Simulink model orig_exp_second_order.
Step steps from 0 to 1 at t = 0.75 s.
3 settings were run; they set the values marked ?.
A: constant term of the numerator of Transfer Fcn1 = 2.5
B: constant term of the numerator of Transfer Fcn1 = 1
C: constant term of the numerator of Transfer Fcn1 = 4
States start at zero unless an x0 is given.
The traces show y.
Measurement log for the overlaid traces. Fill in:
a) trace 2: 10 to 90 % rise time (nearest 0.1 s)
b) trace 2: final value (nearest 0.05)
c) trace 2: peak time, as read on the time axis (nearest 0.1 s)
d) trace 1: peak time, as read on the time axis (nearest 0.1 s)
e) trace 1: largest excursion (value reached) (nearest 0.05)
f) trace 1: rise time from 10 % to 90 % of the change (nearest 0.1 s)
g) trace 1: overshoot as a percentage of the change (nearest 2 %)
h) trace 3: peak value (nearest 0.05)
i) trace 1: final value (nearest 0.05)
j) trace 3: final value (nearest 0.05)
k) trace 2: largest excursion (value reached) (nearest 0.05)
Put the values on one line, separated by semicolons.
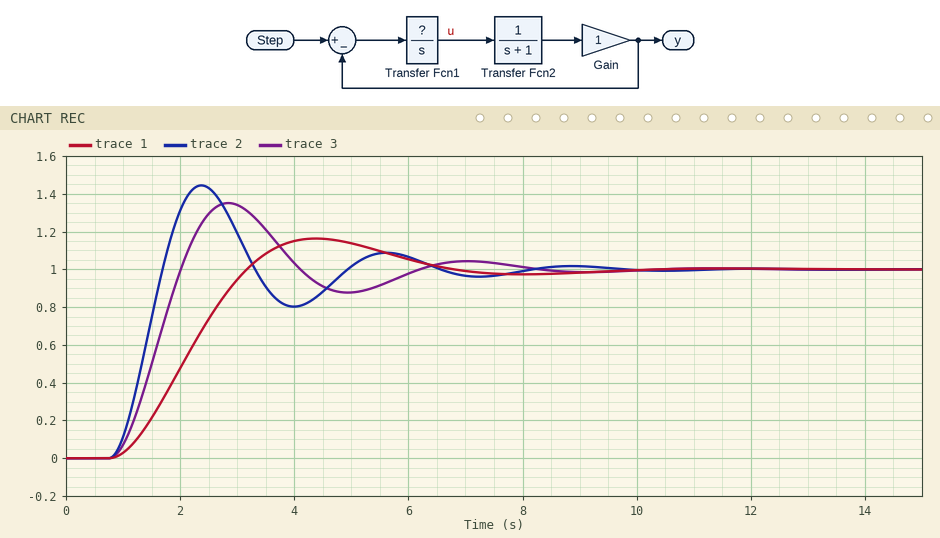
0.6 s; 1.00; 2.4 s; 4.4 s; 1.15; 1.6 s; 16 %; 1.35; 1.00; 1.00; 1.45
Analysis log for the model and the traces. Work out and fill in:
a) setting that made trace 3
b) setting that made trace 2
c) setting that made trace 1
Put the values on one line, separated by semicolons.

A; C; B
